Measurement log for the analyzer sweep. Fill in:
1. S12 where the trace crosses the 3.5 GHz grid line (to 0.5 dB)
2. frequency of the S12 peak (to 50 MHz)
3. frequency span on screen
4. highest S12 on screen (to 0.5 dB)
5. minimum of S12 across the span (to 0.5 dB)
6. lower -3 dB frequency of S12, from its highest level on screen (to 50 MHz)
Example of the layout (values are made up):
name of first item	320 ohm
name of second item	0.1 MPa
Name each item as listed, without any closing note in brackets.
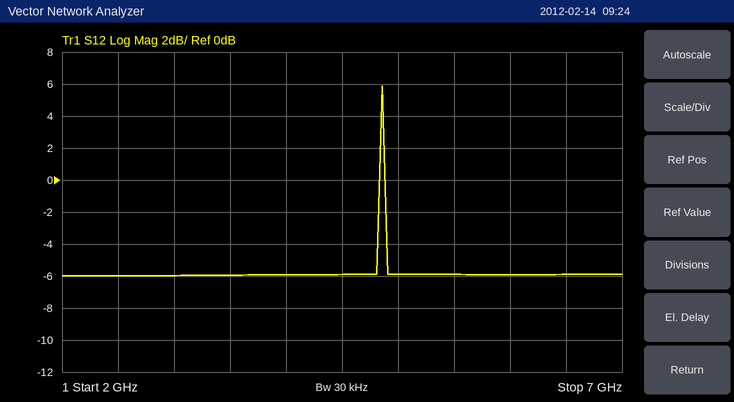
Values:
S12 where the trace crosses the 3.5 GHz grid line	-6.0 dB
frequency of the S12 peak	4.85 GHz
frequency span on screen	5 GHz
highest S12 on screen	6.0 dB
minimum of S12 across the span	-6.0 dB
lower -3 dB frequency of S12, from its highest level on screen	4.85 GHz
